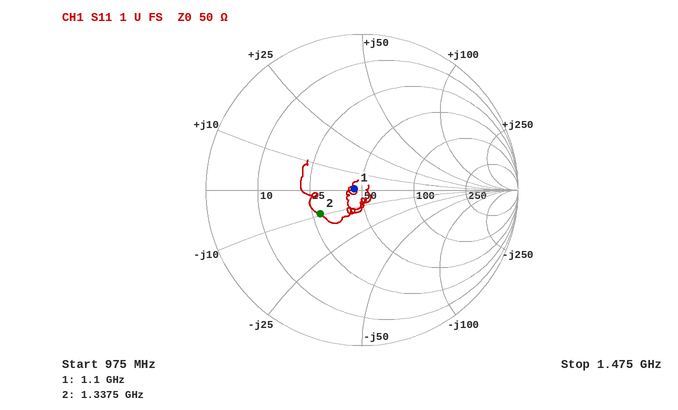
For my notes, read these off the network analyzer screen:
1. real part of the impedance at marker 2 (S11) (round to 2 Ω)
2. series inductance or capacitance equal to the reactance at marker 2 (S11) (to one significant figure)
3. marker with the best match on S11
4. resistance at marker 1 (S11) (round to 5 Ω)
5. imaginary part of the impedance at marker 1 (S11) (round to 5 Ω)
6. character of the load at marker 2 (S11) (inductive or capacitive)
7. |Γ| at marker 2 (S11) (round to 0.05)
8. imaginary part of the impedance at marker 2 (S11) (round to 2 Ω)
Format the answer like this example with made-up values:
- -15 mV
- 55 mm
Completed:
- 28 Ω
- 10 pF
- marker 1
- 45 Ω
- 0 Ω
- capacitive
- 0.30
- -10 Ω
